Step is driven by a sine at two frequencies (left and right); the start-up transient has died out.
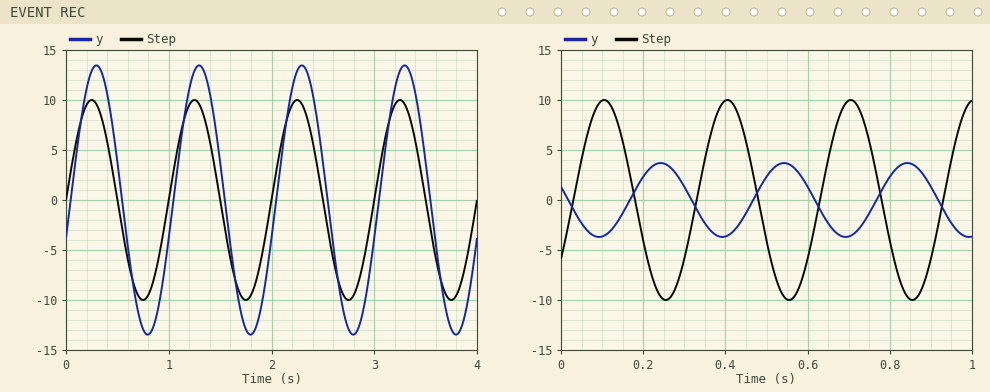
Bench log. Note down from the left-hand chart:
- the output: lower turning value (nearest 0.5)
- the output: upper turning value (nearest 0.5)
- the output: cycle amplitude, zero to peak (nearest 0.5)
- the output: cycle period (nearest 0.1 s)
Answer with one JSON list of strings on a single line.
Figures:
["-13.5", "13.5", "13.5", "1.0 s"]
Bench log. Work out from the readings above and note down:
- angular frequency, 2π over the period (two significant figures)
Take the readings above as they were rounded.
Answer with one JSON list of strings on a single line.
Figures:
["6.3 rad/s"]
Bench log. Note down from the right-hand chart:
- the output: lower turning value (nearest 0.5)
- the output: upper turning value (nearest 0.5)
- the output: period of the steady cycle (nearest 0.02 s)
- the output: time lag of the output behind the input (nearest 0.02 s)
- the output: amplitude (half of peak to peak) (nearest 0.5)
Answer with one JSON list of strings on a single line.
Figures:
["-3.5", "3.5", "0.30 s", "0.14 s", "3.5"]
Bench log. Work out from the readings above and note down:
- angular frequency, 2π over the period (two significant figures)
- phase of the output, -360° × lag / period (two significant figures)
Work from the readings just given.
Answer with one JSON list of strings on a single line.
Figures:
["21 rad/s", "-170°"]
